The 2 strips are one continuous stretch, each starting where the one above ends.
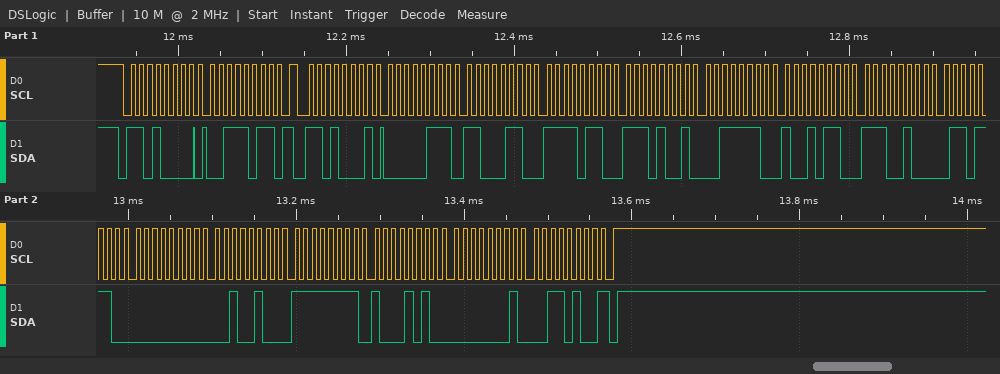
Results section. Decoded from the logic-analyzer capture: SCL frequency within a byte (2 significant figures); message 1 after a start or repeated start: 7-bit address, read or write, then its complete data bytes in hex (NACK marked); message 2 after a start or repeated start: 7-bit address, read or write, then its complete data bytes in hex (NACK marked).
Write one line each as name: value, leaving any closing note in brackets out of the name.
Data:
SCL frequency within a byte: 100 kHz
message 1 after a start or repeated start: 7-bit address, read or write, then its complete data bytes in hex: 0x68 write: 3B
message 2 after a start or repeated start: 7-bit address, read or write, then its complete data bytes in hex: 0x68 read: 07 C6 F6 E9 3E 96 E4 6E 00 24 FF 8A 01 34 NACK
